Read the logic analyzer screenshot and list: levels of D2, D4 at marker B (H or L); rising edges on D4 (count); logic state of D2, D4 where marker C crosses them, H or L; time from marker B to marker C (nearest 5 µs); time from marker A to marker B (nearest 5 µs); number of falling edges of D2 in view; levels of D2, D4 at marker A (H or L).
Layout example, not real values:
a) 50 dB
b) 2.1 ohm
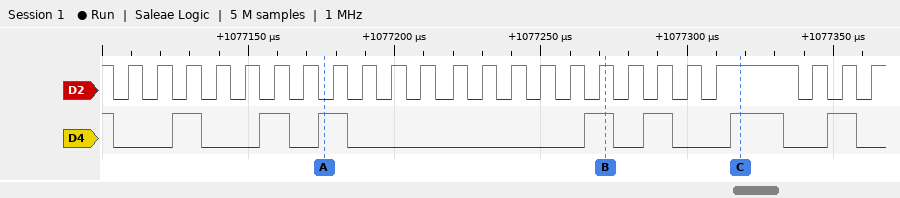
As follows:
a) D2=H, D4=H
b) 7
c) D2=H, D4=H
d) 45 µs
e) 95 µs
f) 24
g) D2=L, D4=H
